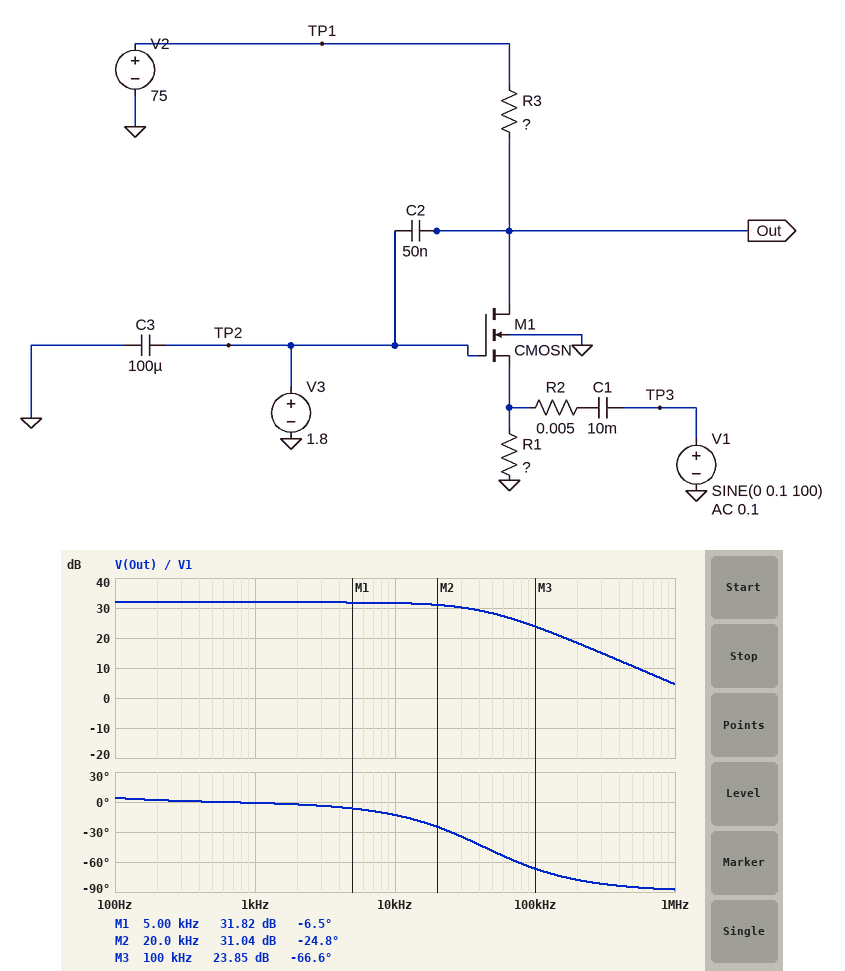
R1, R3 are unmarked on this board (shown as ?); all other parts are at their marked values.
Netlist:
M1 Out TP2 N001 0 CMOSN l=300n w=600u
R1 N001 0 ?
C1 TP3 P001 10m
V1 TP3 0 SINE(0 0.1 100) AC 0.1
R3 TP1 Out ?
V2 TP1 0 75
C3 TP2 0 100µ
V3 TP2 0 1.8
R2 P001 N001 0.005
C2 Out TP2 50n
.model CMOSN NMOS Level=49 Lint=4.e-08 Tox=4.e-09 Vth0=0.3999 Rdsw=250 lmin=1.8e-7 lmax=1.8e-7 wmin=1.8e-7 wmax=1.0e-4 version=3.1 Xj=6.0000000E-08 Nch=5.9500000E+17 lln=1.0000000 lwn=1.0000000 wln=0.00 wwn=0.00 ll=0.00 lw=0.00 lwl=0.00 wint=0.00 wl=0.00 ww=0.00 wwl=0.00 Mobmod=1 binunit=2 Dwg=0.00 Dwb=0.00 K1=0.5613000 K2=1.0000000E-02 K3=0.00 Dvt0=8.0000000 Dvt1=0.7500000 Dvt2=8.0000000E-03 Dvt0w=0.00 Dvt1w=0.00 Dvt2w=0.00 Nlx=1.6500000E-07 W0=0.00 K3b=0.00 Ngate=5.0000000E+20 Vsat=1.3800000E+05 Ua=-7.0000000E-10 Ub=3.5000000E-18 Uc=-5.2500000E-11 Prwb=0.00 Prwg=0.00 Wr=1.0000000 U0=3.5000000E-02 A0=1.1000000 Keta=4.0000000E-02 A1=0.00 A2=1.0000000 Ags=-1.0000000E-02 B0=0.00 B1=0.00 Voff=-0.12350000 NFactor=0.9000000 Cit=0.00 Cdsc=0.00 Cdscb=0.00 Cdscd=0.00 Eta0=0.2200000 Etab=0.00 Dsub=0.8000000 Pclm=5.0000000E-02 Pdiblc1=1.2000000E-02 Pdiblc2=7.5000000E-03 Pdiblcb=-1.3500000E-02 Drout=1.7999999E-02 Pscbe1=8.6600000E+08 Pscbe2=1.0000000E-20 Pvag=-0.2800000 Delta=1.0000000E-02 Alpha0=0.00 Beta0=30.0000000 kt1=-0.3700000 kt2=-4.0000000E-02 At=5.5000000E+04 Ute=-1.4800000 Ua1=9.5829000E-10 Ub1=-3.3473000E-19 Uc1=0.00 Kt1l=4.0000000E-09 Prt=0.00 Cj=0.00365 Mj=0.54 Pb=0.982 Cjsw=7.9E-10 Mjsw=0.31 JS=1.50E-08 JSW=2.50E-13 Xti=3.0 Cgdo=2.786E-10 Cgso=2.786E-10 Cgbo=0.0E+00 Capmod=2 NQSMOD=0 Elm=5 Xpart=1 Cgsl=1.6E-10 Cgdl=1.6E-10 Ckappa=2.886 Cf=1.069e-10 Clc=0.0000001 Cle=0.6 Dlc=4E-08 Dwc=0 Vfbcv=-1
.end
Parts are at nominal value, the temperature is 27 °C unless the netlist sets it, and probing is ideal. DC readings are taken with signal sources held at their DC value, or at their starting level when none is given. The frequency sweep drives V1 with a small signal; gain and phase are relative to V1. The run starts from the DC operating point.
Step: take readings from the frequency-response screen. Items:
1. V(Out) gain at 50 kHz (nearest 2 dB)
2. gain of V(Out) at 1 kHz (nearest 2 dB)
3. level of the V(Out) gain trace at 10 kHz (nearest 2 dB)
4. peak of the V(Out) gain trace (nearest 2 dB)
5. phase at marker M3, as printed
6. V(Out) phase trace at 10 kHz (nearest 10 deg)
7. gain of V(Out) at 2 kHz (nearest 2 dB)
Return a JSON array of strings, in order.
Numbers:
["28 dB", "32 dB", "32 dB", "32 dB", "-66.6 deg", "-10 deg", "32 dB"]
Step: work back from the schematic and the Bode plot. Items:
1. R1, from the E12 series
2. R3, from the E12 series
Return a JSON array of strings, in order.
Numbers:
["3.3 Ω", "220 Ω"]
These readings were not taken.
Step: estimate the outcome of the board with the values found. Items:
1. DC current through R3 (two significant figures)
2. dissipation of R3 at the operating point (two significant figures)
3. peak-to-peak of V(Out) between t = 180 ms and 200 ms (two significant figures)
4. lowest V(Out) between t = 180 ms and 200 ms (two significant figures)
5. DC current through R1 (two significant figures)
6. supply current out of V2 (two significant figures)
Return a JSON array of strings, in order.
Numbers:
["220 mA", "10 W", "7.9 V", "24 V", "220 mA", "220 mA"]
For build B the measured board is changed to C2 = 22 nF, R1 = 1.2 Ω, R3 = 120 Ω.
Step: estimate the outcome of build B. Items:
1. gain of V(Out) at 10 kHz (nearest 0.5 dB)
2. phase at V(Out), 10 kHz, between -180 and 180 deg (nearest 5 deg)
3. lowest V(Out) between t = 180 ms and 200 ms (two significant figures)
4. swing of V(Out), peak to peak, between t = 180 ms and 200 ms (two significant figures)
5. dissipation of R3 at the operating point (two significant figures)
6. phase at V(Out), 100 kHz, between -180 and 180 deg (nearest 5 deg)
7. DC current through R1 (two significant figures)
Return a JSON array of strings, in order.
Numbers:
["28.0 dB", "-5 deg", "27 V", "5.0 V", "17 W", "-35 deg", "380 mA"]
